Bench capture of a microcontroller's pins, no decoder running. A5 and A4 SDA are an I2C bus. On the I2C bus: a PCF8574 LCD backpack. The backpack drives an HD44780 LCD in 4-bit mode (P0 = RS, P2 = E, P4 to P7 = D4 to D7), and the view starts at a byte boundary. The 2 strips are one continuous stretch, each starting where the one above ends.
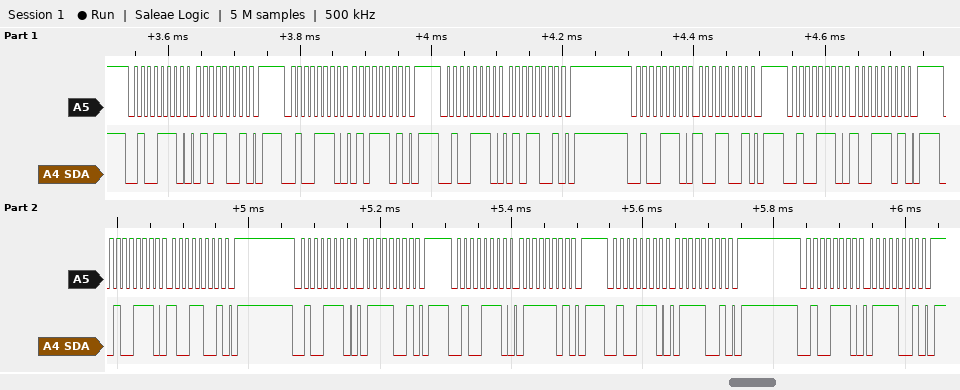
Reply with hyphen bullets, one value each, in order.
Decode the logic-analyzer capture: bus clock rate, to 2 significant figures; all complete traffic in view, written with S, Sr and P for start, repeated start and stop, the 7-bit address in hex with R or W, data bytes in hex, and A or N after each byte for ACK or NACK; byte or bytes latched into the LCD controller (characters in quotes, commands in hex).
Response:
- 100 kHz
- S 27W A 59 A P S 27W A 5D A P S 27W A 59 A P S 27W A 99 A P S 27W A 9D A P S 27W A 99 A P S 27W A 79 A P S 27W A 7D A P S 27W A 79 A P S 27W A 79 A P
- 'Y'
